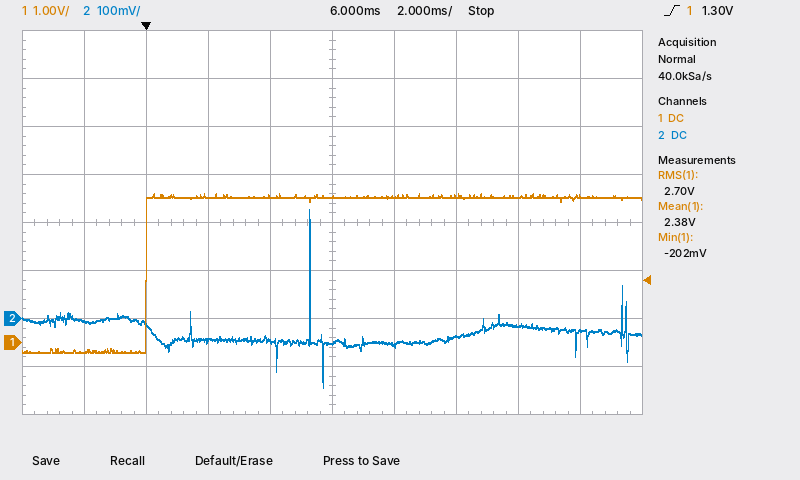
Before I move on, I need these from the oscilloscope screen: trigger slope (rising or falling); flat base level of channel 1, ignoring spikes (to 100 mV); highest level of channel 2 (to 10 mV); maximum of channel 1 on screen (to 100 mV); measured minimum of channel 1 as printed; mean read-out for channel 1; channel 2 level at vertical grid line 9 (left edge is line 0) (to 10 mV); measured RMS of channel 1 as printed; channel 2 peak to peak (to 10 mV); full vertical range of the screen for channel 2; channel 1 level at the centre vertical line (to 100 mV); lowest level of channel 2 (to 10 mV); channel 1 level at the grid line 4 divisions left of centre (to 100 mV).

rising
-200 mV
230 mV
3.1 V
-202 mV
2.38 V
-30 mV
2.70 V
370 mV
800 mV
3.0 V
-140 mV
-200 mV
